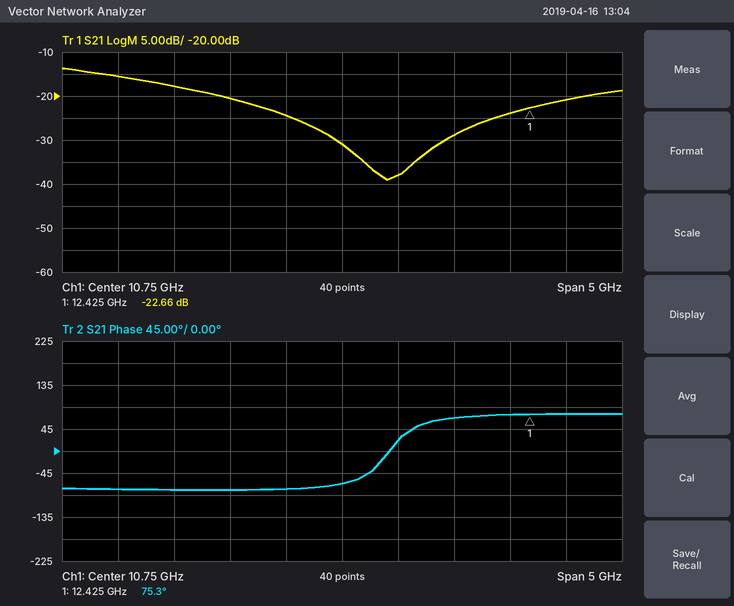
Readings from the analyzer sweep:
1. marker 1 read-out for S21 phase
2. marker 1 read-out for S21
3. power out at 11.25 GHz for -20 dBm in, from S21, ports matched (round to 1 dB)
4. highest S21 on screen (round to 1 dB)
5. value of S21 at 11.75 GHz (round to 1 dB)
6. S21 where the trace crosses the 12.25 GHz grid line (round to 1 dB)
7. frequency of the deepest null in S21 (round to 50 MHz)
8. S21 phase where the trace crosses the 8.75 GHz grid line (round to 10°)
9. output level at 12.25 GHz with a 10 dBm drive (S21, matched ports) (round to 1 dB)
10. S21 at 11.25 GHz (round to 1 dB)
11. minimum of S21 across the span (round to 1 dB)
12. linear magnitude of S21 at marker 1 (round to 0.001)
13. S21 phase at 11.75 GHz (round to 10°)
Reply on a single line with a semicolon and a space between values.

75.3°; -22.66 dB; -58 dBm; -14 dB; -29 dB; -24 dB; 11.15 GHz; -80°; -14 dBm; -38 dB; -39 dB; 0.074; 70°
